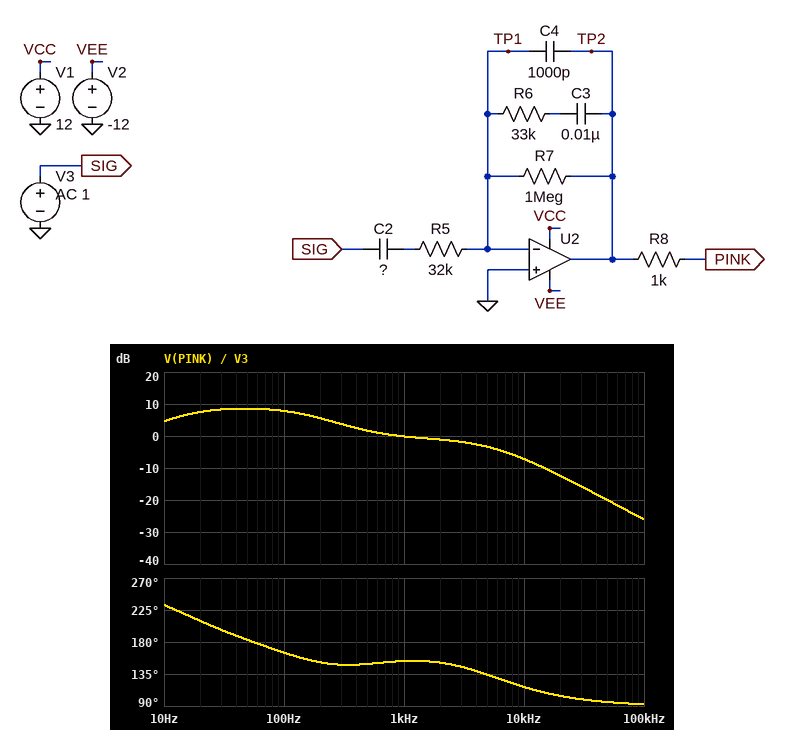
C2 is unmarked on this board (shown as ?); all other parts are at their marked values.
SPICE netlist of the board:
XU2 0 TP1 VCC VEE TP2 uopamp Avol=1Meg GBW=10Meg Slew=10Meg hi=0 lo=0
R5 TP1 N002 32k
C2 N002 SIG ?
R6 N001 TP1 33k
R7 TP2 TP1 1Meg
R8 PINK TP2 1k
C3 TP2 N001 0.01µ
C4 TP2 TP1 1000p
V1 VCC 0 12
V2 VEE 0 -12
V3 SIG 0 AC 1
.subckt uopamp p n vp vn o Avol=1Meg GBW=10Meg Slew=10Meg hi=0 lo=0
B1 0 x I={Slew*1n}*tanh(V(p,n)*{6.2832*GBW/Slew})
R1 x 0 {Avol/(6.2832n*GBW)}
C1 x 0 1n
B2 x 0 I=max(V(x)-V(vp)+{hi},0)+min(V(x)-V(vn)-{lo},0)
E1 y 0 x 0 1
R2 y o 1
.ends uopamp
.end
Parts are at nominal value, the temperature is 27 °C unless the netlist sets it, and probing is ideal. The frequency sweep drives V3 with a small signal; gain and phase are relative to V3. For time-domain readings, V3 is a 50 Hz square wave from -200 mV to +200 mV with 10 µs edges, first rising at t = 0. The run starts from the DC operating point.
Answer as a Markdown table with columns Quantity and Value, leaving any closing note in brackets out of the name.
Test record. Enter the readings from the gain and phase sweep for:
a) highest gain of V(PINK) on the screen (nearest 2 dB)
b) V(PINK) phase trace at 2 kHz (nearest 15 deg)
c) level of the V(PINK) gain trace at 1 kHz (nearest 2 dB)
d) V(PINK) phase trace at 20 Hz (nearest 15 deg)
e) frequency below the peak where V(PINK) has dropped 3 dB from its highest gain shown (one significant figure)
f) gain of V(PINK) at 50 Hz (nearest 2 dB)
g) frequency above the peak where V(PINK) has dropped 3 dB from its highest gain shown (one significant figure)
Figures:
| Quantity | Value |
|---|---|
| highest gain of V(PINK) on the screen | 8 dB |
| V(PINK) phase trace at 2 kHz | 150 deg |
| level of the V(PINK) gain trace at 1 kHz | 0 dB |
| V(PINK) phase trace at 20 Hz | 210 deg |
| frequency below the peak where V(PINK) has dropped 3 dB from its highest gain shown | 10 Hz |
| gain of V(PINK) at 50 Hz | 8 dB |
| frequency above the peak where V(PINK) has dropped 3 dB from its highest gain shown | 200 Hz |
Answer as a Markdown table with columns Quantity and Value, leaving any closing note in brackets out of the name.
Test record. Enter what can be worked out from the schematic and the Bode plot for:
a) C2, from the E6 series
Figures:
| Quantity | Value |
|---|---|
| C2, from the E6 series | 33 nF |
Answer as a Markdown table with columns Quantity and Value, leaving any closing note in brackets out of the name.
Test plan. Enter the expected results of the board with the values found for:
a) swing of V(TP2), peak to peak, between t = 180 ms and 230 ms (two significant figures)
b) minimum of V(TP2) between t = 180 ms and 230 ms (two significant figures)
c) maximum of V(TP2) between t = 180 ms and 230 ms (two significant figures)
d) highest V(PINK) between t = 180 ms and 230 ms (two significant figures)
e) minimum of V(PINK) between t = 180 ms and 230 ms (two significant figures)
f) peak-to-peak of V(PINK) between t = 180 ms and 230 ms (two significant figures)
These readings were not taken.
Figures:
| Quantity | Value |
|---|---|
| swing of V(TP2), peak to peak, between t = 180 ms and 230 ms | 1.3 V |
| minimum of V(TP2) between t = 180 ms and 230 ms | -630 mV |
| maximum of V(TP2) between t = 180 ms and 230 ms | 630 mV |
| highest V(PINK) between t = 180 ms and 230 ms | 630 mV |
| minimum of V(PINK) between t = 180 ms and 230 ms | -630 mV |
| peak-to-peak of V(PINK) between t = 180 ms and 230 ms | 1.3 V |
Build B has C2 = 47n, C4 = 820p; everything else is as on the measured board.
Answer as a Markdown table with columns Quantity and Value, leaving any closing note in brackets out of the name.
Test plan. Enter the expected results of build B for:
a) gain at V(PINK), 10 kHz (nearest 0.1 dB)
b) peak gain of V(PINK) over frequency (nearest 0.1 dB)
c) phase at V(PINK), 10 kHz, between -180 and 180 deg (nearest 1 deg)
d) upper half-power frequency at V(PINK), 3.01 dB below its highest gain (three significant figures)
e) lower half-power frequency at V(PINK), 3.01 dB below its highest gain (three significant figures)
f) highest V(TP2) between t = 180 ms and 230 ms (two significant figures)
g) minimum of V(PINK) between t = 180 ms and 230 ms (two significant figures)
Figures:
| Quantity | Value |
|---|---|
| gain at V(PINK), 10 kHz | -5.9 dB |
| peak gain of V(PINK) over frequency | 11.4 dB |
| phase at V(PINK), 10 kHz, between -180 and 180 deg | 121 deg |
| upper half-power frequency at V(PINK), 3.01 dB below its highest gain | 140 Hz |
| lower half-power frequency at V(PINK), 3.01 dB below its highest gain | 11.6 Hz |
| highest V(TP2) between t = 180 ms and 230 ms | 840 mV |
| minimum of V(PINK) between t = 180 ms and 230 ms | -840 mV |
